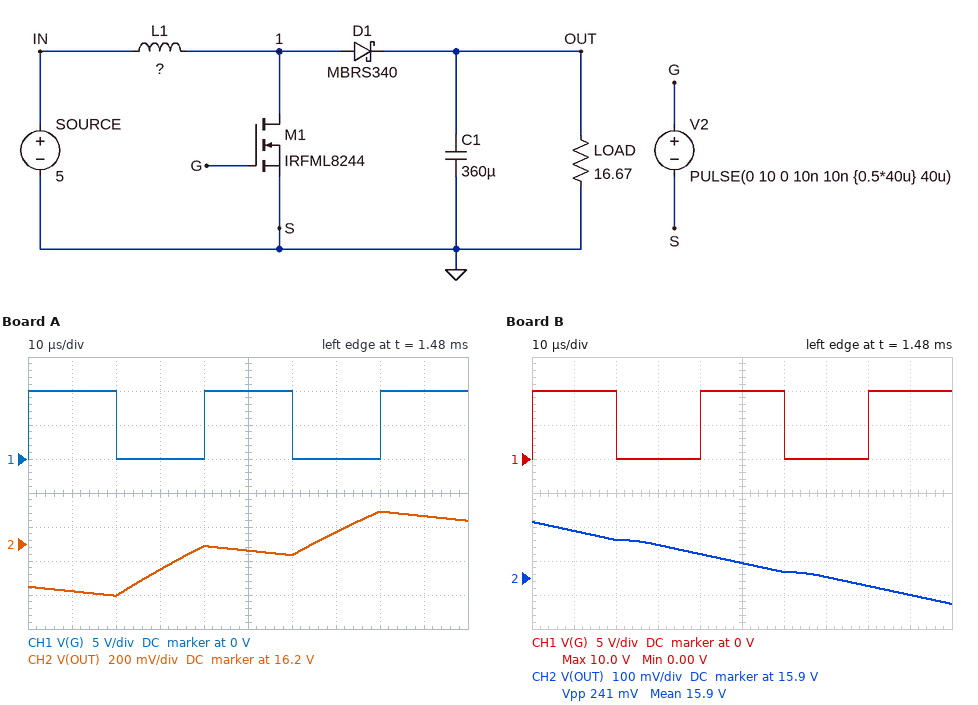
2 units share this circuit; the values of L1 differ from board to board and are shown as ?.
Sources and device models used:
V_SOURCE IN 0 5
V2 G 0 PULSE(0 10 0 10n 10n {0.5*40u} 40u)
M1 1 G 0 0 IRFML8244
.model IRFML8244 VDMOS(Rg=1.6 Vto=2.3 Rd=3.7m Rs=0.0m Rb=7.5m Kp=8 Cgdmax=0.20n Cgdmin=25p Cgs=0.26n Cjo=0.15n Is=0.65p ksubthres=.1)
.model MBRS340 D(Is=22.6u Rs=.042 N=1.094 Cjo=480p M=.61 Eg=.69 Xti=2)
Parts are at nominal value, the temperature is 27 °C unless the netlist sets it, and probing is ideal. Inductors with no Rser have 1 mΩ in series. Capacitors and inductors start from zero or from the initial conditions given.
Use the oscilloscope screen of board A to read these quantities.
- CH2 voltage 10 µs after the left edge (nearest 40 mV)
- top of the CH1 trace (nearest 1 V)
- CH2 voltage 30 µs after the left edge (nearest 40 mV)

15.92 V
10 V
16.04 V
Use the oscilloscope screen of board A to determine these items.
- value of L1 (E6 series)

220 µH
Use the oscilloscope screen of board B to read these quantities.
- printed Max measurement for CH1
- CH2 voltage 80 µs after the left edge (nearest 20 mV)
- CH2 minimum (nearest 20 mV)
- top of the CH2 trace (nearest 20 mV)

10.0 V
15.88 V
15.82 V
16.06 V
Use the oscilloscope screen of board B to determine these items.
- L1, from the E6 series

100 µH
